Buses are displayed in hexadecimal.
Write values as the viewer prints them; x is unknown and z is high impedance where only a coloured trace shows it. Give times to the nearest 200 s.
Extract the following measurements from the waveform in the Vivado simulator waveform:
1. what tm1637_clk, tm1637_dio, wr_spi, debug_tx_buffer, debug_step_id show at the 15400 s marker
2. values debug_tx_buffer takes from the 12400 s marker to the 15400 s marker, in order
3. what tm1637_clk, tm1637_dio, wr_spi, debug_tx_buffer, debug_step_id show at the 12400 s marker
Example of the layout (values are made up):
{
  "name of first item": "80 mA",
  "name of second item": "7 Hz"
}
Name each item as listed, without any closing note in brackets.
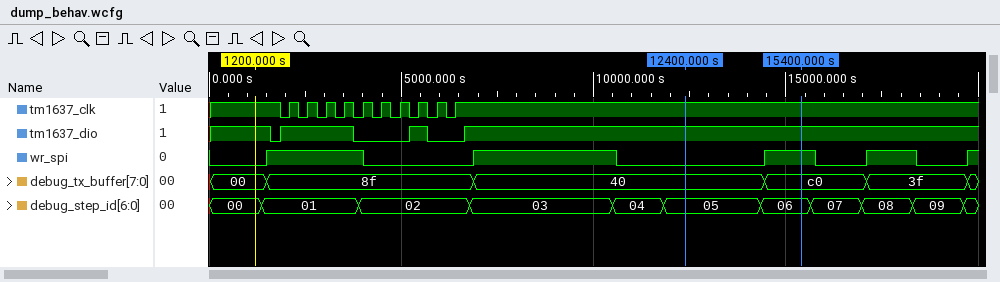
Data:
{
  "what tm1637_clk, tm1637_dio, wr_spi, debug_tx_buffer, debug_step_id show at the 15400 s marker": "tm1637_clk=1, tm1637_dio=1, wr_spi=1, debug_tx_buffer=c0, debug_step_id=06",
  "values debug_tx_buffer takes from the 12400 s marker to the 15400 s marker, in order": "40, c0",
  "what tm1637_clk, tm1637_dio, wr_spi, debug_tx_buffer, debug_step_id show at the 12400 s marker": "tm1637_clk=1, tm1637_dio=1, wr_spi=0, debug_tx_buffer=40, debug_step_id=05"
}
